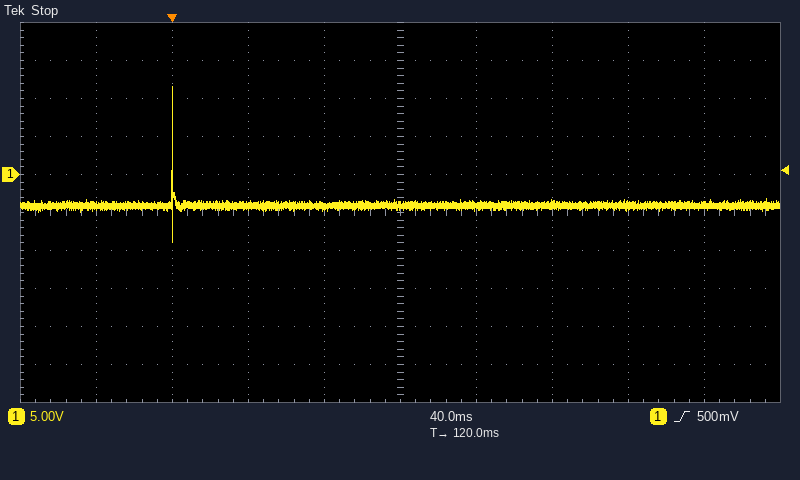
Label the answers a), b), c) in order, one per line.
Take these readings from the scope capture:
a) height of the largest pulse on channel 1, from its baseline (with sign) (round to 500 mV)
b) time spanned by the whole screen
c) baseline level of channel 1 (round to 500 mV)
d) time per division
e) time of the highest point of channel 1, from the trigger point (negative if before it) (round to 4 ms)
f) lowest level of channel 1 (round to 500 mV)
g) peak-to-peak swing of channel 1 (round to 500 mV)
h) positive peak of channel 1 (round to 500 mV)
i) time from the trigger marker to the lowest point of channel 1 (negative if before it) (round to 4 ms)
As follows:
a) +15.5 V
b) 400 ms
c) -4.0 V
d) 40 ms
e) 0 ms
f) -9.0 V
g) 20.5 V
h) 11.5 V
i) 0 ms
